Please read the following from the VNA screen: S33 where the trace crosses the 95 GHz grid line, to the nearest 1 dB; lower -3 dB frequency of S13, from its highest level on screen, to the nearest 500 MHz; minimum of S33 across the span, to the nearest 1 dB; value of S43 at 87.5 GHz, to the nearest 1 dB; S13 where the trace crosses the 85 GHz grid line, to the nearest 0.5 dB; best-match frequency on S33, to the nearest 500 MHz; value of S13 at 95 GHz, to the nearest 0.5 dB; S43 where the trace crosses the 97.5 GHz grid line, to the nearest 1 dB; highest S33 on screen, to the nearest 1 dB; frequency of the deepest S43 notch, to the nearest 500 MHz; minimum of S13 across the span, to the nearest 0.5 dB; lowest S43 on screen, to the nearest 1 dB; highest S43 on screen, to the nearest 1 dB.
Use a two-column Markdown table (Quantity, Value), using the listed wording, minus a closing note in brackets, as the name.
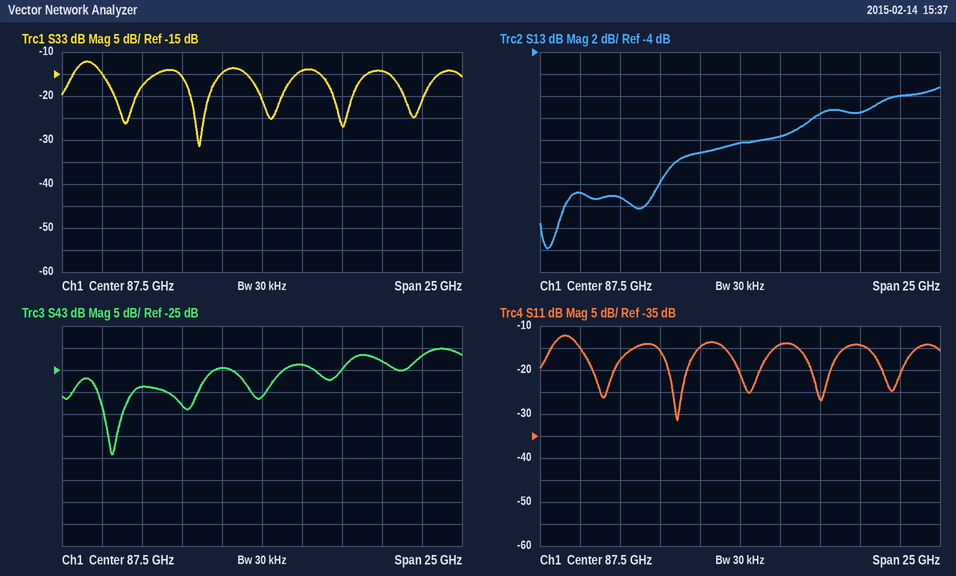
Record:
| Quantity | Value |
|---|---|
| S33 where the trace crosses the 95 GHz grid line, to the nearest 1 dB | -14 dB |
| lower -3 dB frequency of S13, from its highest level on screen, to the nearest 500 MHz | 92.0 GHz |
| minimum of S33 across the span, to the nearest 1 dB | -31 dB |
| value of S43 at 87.5 GHz, to the nearest 1 dB | -31 dB |
| S13 where the trace crosses the 85 GHz grid line, to the nearest 0.5 dB | -13.0 dB |
| best-match frequency on S33, to the nearest 500 MHz | 83.5 GHz |
| value of S13 at 95 GHz, to the nearest 0.5 dB | -9.5 dB |
| S43 where the trace crosses the 97.5 GHz grid line, to the nearest 1 dB | -22 dB |
| highest S33 on screen, to the nearest 1 dB | -12 dB |
| frequency of the deepest S43 notch, to the nearest 500 MHz | 78.0 GHz |
| minimum of S13 across the span, to the nearest 0.5 dB | -22.0 dB |
| lowest S43 on screen, to the nearest 1 dB | -44 dB |
| highest S43 on screen, to the nearest 1 dB | -20 dB |
